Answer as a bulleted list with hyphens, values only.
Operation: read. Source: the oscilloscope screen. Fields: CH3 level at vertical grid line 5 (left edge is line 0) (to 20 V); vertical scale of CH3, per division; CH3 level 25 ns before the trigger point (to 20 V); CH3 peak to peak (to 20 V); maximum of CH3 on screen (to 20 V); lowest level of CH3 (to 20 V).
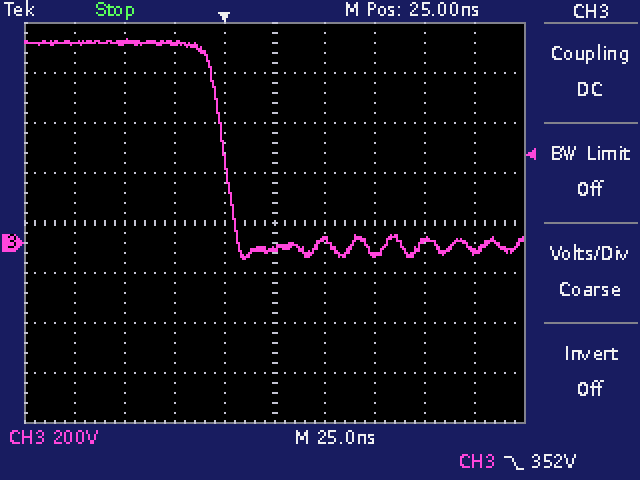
- -20 V
- 200 V
- 800 V
- 880 V
- 820 V
- -60 V
